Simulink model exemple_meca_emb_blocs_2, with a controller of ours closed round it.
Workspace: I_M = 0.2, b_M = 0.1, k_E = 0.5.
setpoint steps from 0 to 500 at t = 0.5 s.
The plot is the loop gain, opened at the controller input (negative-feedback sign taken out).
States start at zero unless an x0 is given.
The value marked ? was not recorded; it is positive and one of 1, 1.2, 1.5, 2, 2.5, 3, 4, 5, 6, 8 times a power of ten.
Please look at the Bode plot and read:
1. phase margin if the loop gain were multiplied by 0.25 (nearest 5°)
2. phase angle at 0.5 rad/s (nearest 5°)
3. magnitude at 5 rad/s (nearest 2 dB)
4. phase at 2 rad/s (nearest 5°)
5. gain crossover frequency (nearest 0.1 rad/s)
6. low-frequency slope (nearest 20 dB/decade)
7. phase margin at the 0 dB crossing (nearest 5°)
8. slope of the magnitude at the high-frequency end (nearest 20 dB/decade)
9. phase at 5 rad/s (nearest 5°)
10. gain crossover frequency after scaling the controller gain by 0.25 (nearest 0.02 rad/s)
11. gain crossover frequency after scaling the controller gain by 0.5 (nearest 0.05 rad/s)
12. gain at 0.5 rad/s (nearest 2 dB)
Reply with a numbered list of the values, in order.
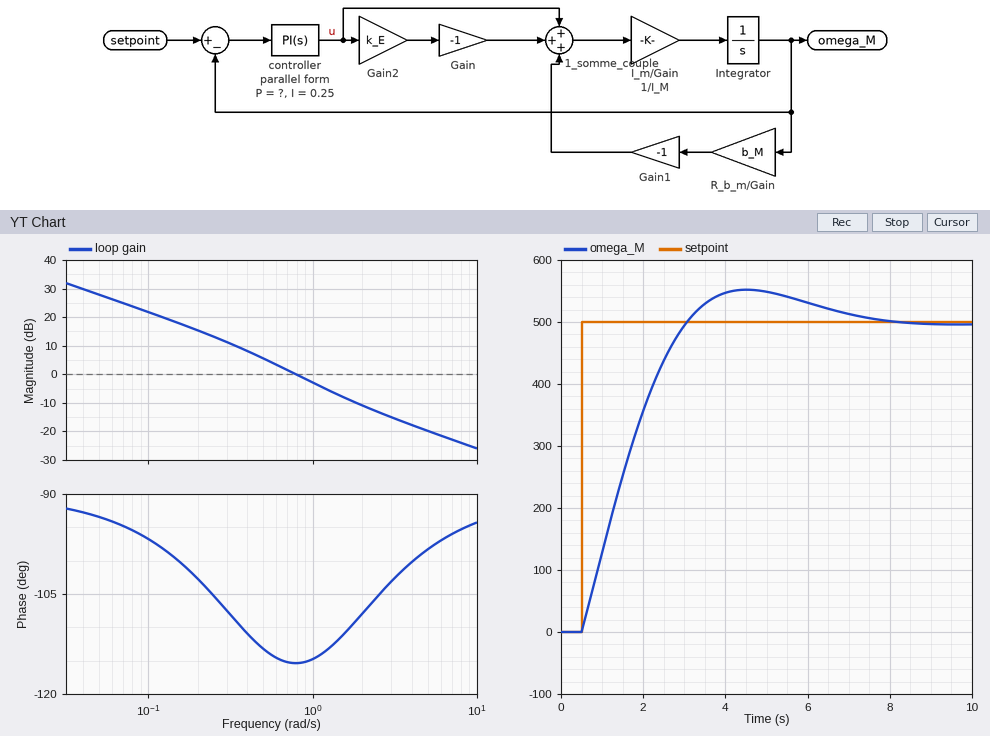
1. 75°
2. -115°
3. -20 dB
4. -110°
5. 0.8 rad/s
6. -20 dB/decade
7. 65°
8. -20 dB/decade
9. -100°
10. 0.28 rad/s
11. 0.50 rad/s
12. 6 dB
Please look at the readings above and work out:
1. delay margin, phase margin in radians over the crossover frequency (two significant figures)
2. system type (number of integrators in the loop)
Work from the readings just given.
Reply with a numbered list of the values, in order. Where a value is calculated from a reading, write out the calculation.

1. 65 × π / 180 / 0.8 = 1.4 s
2. 1
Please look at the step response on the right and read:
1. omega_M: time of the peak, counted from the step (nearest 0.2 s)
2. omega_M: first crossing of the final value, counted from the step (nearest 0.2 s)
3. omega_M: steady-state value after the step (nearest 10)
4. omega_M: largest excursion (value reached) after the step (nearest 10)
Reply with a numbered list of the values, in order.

1. 4.0 s
2. 2.6 s
3. 500
4. 550
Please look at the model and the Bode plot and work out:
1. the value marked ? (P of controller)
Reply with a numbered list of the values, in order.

1. 0.2
